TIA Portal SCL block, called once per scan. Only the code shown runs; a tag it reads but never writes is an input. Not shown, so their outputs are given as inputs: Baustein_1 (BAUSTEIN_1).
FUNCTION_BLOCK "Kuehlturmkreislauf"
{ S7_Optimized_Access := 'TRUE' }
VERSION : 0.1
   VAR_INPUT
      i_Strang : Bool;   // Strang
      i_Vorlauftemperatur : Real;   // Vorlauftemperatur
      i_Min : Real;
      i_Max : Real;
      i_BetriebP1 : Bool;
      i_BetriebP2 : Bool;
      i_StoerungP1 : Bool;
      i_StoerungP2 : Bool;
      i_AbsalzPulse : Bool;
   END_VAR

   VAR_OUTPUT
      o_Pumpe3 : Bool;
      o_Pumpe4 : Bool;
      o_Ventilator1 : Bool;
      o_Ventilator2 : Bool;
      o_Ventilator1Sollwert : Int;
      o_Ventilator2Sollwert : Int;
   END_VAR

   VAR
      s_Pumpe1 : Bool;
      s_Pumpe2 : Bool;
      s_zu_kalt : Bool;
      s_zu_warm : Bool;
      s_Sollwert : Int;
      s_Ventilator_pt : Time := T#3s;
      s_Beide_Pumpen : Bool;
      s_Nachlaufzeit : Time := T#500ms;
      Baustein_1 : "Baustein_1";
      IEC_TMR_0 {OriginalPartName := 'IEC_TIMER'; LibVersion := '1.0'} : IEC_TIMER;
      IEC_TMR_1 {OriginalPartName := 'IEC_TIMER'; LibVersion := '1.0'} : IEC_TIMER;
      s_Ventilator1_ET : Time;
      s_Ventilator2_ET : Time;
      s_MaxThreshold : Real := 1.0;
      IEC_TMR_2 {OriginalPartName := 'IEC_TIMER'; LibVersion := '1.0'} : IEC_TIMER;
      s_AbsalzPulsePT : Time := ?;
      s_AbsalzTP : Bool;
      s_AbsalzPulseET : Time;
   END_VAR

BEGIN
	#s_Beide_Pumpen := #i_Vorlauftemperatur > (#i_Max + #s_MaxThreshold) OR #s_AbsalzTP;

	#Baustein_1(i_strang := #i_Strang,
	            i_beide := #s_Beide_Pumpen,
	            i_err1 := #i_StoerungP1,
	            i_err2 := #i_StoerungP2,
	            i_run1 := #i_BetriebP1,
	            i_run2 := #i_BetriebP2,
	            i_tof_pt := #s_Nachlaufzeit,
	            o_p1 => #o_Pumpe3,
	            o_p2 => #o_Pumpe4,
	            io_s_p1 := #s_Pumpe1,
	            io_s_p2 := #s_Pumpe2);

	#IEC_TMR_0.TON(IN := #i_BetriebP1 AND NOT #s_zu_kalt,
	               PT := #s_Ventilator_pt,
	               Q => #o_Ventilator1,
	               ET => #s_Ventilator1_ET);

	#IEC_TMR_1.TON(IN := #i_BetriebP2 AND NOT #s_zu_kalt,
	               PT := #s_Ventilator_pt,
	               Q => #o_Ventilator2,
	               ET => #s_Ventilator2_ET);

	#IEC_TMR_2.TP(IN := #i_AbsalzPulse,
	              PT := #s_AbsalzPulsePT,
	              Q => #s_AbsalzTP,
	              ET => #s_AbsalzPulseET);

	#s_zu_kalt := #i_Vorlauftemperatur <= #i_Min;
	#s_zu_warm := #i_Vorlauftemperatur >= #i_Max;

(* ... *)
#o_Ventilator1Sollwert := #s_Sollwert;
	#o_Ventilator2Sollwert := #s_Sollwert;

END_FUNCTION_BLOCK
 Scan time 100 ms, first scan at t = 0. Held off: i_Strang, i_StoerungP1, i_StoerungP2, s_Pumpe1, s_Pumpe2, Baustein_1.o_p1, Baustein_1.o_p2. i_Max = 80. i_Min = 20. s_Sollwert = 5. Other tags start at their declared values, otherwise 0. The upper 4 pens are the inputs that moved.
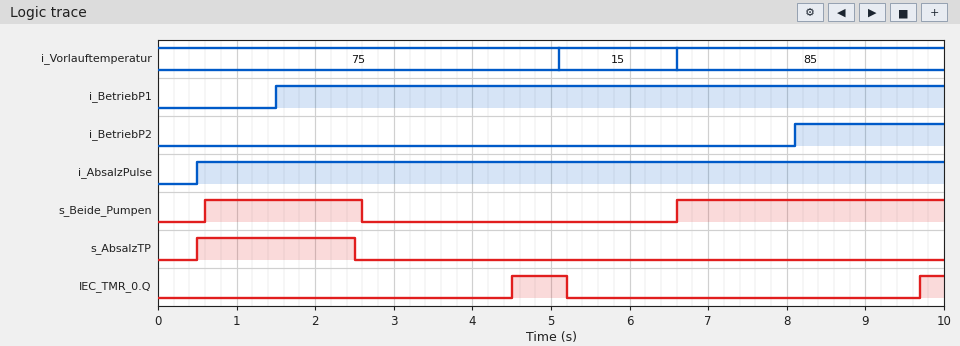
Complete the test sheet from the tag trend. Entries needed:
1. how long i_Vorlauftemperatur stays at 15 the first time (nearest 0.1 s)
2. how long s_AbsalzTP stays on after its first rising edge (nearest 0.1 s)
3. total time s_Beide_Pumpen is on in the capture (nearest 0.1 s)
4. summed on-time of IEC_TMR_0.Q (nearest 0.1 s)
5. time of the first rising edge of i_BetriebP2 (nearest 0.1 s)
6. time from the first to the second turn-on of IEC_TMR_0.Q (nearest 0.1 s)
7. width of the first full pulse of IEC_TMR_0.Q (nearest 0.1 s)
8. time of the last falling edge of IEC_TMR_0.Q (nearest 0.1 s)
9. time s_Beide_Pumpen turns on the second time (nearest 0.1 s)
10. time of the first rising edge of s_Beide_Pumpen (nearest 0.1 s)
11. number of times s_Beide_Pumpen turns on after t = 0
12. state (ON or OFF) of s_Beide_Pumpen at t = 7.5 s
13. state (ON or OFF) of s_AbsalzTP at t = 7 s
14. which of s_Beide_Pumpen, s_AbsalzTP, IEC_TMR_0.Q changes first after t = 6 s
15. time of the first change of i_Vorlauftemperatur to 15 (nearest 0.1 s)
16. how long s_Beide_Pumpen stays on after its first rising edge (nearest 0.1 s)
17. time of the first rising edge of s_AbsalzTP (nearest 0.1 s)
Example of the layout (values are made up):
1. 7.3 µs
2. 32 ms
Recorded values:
1. 1.5 s
2. 2.0 s
3. 5.4 s
4. 1.0 s
5. 8.1 s
6. 5.2 s
7. 0.7 s
8. 5.2 s
9. 6.6 s
10. 0.6 s
11. 2
12. ON
13. OFF
14. s_Beide_Pumpen
15. 5.1 s
16. 2.0 s
17. 0.5 s
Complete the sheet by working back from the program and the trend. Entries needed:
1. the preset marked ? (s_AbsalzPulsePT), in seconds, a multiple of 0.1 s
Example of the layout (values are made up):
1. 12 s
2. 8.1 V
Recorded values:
1. 2.0 s
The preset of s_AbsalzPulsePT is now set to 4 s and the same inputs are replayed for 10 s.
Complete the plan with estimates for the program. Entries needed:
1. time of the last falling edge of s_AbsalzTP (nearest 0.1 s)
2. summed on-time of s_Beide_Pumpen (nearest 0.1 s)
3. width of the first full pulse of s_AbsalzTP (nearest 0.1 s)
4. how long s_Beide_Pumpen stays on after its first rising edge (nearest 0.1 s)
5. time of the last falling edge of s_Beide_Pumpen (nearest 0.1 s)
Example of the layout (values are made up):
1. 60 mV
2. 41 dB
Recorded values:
1. 4.5 s
2. 7.4 s
3. 4.0 s
4. 4.0 s
5. 4.6 s
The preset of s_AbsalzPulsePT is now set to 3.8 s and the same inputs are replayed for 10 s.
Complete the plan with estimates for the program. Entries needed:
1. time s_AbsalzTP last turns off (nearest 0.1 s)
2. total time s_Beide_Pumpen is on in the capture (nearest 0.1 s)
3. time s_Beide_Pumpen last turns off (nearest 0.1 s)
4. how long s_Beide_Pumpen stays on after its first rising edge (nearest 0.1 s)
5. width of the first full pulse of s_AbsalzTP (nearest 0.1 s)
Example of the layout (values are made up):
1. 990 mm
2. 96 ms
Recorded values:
1. 4.3 s
2. 7.2 s
3. 4.4 s
4. 3.8 s
5. 3.8 s
